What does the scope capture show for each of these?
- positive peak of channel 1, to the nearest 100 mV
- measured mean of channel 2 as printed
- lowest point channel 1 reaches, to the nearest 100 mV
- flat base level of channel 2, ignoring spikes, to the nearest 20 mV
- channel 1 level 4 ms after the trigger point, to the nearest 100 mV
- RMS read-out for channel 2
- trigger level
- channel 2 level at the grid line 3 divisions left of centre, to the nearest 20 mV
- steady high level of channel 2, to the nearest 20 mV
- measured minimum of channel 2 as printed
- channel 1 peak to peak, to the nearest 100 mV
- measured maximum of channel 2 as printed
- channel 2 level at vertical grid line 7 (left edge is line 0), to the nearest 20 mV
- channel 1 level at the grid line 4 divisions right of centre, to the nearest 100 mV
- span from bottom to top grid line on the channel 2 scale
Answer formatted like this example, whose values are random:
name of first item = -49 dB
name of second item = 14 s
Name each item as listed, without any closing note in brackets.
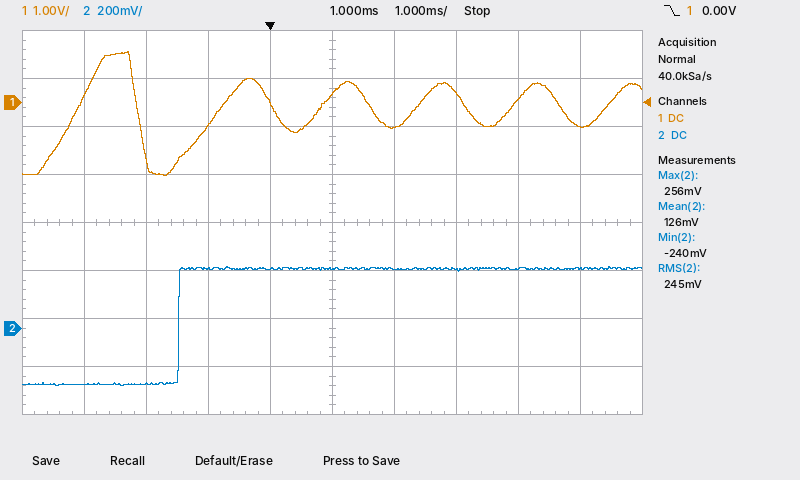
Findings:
positive peak of channel 1, to the nearest 100 mV = 1.1 V
measured mean of channel 2 as printed = 126 mV
lowest point channel 1 reaches, to the nearest 100 mV = -1.5 V
flat base level of channel 2, ignoring spikes, to the nearest 20 mV = -240 mV
channel 1 level 4 ms after the trigger point, to the nearest 100 mV = 100 mV
RMS read-out for channel 2 = 245 mV
trigger level = 0.00 V
channel 2 level at the grid line 3 divisions left of centre, to the nearest 20 mV = -240 mV
steady high level of channel 2, to the nearest 20 mV = 240 mV
measured minimum of channel 2 as printed = -240 mV
channel 1 peak to peak, to the nearest 100 mV = 2.6 V
measured maximum of channel 2 as printed = 256 mV
channel 2 level at vertical grid line 7 (left edge is line 0), to the nearest 20 mV = 240 mV
channel 1 level at the grid line 4 divisions right of centre, to the nearest 100 mV = -500 mV
span from bottom to top grid line on the channel 2 scale = 1.6 V
